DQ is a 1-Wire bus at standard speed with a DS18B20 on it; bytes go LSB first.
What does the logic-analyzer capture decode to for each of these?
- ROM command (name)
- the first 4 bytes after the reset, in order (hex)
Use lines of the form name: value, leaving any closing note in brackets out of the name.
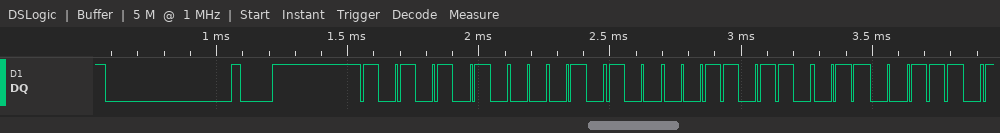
ROM command: Match ROM
the first 4 bytes after the reset, in order: 55 28 6C E6
